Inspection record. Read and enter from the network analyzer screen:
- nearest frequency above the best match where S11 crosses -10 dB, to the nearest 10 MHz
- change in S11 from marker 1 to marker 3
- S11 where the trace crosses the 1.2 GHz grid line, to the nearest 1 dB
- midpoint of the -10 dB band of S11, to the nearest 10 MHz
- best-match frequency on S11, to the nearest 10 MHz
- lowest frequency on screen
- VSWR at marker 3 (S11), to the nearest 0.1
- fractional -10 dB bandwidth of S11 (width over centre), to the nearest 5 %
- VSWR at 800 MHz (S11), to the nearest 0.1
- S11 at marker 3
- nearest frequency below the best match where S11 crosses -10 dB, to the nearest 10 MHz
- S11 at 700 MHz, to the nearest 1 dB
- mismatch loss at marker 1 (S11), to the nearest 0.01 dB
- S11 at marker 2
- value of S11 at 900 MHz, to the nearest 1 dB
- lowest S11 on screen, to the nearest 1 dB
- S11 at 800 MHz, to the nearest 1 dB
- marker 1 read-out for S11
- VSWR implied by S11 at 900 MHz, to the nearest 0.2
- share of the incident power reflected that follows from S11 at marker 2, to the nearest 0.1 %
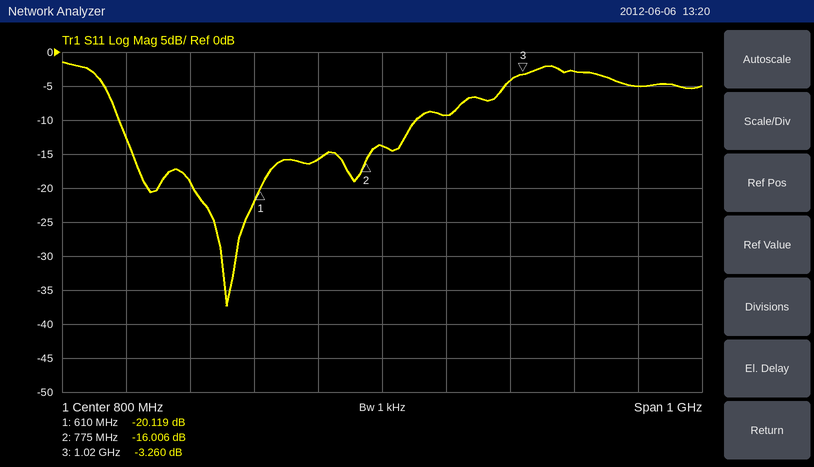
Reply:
850 MHz
16.859 dB
-5 dB
620 MHz
560 MHz
300 MHz
5.4
75 %
1.5
-3.260 dB
390 MHz
-16 dB
0.04 dB
-16.006 dB
-9 dB
-37 dB
-14 dB
-20.119 dB
2.0
2.5 %
